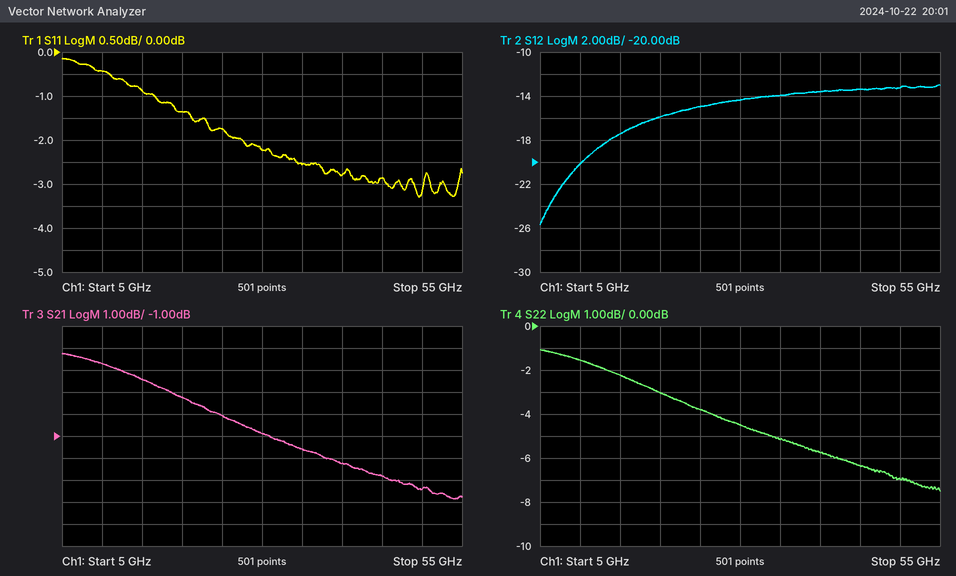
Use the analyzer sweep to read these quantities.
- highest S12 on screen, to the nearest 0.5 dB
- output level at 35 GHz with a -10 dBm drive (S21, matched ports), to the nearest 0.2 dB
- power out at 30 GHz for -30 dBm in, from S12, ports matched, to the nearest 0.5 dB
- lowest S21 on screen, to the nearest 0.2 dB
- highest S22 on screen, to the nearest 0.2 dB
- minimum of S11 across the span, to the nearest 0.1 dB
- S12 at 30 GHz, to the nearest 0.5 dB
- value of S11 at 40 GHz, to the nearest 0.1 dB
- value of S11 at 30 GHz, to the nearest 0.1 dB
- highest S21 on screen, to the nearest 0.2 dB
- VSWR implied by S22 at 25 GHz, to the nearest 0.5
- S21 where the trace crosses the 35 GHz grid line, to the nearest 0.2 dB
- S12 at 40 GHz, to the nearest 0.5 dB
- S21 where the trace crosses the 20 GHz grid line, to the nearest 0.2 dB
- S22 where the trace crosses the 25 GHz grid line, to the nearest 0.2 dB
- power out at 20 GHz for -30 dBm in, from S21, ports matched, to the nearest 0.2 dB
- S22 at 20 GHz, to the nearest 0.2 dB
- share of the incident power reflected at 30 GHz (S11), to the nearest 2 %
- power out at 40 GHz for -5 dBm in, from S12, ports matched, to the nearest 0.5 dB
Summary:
-13.0 dB
-11.6 dBm
-44.5 dBm
-3.8 dB
-1.0 dB
-3.3 dB
-14.5 dB
-2.8 dB
-2.2 dB
2.8 dB
4.5
-1.6 dB
-13.5 dB
0.8 dB
-3.8 dB
-29.2 dBm
-3.0 dB
60 %
-18.5 dBm
